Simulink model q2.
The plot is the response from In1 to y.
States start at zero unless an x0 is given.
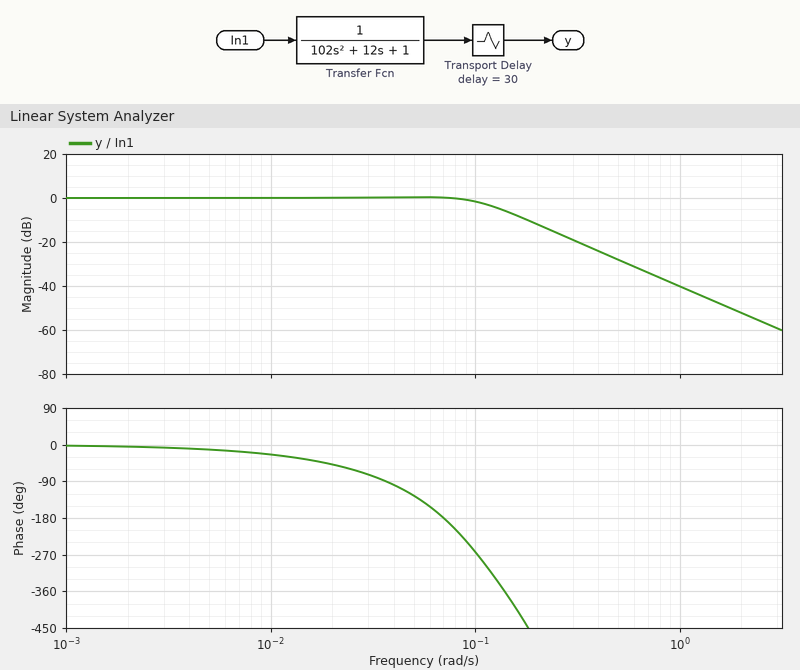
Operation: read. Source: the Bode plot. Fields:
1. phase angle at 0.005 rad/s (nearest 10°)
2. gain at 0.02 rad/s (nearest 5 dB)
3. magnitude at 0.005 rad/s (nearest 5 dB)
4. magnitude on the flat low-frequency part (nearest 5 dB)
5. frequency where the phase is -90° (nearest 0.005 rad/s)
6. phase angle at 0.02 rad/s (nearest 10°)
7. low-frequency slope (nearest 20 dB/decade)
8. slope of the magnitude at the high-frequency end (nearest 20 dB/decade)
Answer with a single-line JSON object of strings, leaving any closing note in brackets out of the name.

{"phase angle at 0.005 rad/s": "-10°", "gain at 0.02 rad/s": "0 dB", "magnitude at 0.005 rad/s": "0 dB", "magnitude on the flat low-frequency part": "0 dB", "frequency where the phase is -90°": "0.035 rad/s", "phase angle at 0.02 rad/s": "-50°", "low-frequency slope": "0 dB/decade", "slope of the magnitude at the high-frequency end": "-40 dB/decade"}
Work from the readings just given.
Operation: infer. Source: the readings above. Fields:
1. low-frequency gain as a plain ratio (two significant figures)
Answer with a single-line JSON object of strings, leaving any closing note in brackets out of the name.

{"low-frequency gain as a plain ratio": "1.0"}
